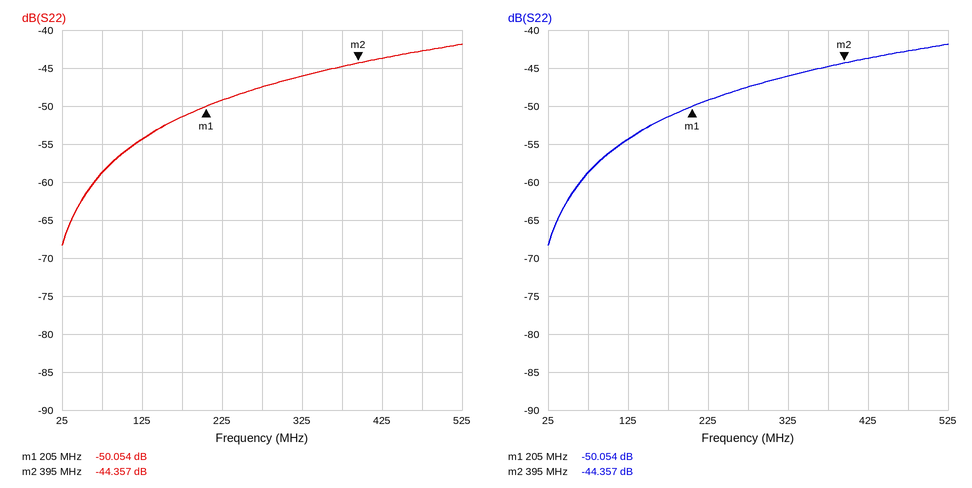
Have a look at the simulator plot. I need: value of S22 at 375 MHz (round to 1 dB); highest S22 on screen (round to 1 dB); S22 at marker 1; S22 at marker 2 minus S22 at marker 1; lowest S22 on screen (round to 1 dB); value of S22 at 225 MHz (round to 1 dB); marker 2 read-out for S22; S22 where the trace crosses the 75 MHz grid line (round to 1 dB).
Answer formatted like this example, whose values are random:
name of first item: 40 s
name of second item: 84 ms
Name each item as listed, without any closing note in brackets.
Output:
value of S22 at 375 MHz: -45 dB
highest S22 on screen: -42 dB
S22 at marker 1: -50.054 dB
S22 at marker 2 minus S22 at marker 1: 5.697 dB
lowest S22 on screen: -68 dB
value of S22 at 225 MHz: -49 dB
marker 2 read-out for S22: -44.357 dB
S22 where the trace crosses the 75 MHz grid line: -59 dB
